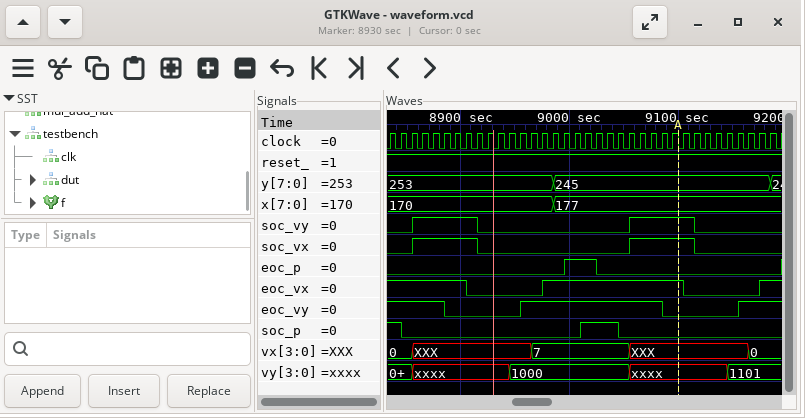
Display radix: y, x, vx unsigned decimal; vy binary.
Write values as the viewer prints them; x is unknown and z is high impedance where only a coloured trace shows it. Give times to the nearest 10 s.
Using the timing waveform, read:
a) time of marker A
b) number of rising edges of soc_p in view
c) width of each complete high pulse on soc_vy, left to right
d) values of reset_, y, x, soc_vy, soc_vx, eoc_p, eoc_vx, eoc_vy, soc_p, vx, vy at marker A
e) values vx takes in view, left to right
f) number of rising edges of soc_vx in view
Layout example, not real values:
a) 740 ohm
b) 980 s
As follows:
a) 9100 s
b) 1
c) 60 s, 60 s
d) reset_=1, y=245, x=177, soc_vy=1, soc_vx=1, eoc_p=0, eoc_vx=1, eoc_vy=0, soc_p=0, vx=XXX, vy=xxxx
e) 0, XXX, 7, XXX, 0
f) 2
